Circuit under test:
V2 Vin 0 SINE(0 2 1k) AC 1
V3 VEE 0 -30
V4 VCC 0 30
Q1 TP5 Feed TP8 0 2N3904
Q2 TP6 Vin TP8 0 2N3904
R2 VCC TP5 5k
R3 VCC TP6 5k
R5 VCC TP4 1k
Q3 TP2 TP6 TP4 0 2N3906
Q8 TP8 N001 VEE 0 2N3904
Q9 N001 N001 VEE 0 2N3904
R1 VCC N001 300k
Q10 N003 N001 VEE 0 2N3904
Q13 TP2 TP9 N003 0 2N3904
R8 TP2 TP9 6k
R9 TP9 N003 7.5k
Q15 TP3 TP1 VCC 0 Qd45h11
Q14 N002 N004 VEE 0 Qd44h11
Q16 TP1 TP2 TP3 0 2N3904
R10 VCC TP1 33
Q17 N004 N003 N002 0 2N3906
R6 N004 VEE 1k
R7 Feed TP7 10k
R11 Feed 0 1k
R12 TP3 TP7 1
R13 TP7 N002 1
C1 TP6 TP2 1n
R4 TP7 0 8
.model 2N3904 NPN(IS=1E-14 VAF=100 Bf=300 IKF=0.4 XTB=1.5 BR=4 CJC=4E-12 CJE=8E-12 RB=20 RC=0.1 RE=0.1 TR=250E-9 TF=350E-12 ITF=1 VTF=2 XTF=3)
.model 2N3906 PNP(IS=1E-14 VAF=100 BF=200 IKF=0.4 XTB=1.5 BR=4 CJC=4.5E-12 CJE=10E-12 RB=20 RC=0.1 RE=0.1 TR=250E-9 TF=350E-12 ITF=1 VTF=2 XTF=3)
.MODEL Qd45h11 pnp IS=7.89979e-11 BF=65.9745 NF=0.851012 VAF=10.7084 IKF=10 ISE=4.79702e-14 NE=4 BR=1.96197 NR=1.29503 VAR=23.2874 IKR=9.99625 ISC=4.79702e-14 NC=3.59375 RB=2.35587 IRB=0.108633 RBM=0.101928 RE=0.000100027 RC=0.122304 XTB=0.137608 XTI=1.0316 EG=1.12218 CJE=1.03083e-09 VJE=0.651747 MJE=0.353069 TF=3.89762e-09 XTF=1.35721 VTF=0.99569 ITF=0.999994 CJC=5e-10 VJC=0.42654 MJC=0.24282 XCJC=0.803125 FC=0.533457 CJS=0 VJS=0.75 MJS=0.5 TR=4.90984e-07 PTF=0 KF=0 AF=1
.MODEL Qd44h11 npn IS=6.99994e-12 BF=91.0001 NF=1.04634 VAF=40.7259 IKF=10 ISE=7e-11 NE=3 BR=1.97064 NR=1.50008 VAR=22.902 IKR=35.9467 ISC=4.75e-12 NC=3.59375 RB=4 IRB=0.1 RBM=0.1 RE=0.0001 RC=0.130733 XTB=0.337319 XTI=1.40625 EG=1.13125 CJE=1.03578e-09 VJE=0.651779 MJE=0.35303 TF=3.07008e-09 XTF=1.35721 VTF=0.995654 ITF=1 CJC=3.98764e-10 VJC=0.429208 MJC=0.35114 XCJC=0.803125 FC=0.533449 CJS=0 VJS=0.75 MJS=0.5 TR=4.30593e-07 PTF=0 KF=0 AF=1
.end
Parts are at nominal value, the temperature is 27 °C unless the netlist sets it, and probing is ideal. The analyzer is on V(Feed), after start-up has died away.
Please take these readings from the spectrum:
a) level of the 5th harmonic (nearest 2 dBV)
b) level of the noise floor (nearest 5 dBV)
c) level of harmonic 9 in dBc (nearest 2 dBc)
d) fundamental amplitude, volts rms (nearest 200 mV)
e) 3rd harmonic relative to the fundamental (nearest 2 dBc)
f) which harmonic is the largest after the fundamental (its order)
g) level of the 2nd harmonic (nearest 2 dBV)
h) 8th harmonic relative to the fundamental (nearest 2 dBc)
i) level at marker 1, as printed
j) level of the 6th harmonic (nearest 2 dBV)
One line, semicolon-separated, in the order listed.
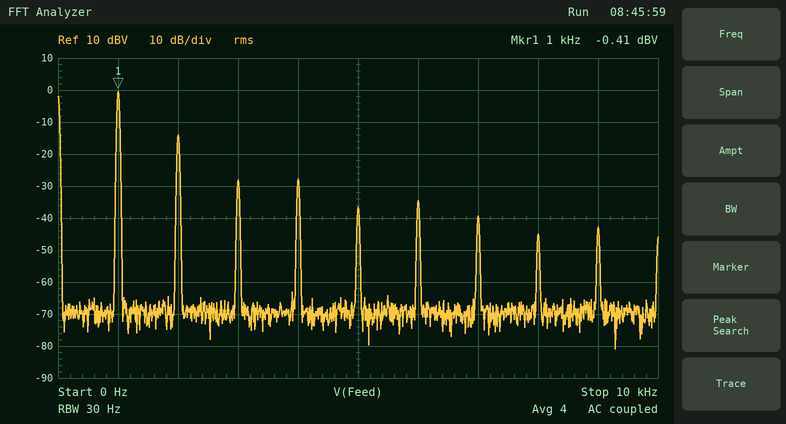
-36 dBV; -70 dBV; -42 dBc; 1.0 V; -28 dBc; 2; -14 dBV; -44 dBc; -0.41 dBV; -34 dBV
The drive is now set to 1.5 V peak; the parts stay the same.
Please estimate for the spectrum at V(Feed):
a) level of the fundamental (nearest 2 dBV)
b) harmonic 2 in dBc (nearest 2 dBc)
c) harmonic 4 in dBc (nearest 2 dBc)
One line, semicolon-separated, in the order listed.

-2 dBV; -16 dBc; -32 dBc
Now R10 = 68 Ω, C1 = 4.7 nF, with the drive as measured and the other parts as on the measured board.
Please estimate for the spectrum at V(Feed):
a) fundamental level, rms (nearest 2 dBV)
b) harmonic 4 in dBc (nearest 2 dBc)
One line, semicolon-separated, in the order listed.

-12 dBV; -24 dBc
